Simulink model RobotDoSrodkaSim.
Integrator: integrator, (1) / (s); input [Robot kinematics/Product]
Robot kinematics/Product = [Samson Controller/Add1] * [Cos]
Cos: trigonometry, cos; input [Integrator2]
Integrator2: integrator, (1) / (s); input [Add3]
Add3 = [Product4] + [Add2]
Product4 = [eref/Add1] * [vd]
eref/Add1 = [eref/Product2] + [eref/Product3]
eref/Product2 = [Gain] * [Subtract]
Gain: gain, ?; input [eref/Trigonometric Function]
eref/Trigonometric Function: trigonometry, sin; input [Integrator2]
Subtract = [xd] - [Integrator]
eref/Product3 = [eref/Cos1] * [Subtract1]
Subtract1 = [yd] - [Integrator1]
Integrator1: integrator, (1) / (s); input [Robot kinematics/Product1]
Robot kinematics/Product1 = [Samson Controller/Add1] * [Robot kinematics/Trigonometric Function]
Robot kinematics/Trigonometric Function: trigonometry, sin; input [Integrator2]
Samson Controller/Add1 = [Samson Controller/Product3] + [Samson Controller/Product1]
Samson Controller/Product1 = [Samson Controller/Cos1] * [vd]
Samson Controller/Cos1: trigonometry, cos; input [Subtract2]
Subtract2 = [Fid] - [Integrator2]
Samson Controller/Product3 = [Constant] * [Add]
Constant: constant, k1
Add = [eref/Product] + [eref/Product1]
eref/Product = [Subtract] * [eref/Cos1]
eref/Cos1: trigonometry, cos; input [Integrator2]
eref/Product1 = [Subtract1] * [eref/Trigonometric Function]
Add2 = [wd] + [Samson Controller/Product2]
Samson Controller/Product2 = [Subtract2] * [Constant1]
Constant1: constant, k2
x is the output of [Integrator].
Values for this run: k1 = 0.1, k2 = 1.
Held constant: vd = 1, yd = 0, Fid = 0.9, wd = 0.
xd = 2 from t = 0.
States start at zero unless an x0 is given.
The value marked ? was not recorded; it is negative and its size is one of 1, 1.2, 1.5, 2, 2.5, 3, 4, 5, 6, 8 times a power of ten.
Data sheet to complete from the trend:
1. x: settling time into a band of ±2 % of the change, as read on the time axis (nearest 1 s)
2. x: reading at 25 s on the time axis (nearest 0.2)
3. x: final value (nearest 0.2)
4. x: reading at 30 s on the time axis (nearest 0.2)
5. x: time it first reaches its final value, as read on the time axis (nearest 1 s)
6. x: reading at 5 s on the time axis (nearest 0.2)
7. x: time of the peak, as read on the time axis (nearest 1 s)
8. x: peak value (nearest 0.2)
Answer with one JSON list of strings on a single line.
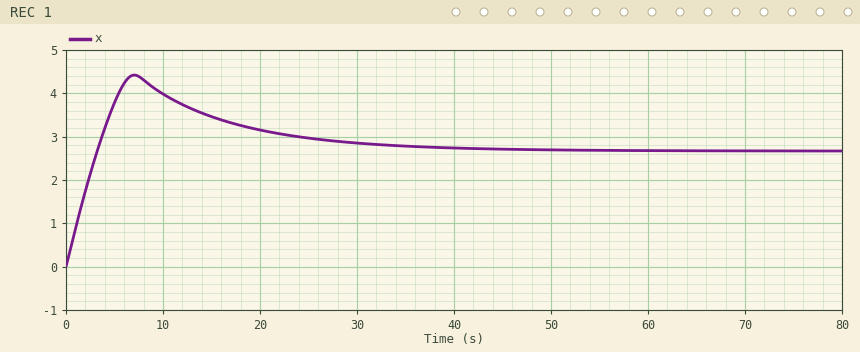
["43 s", "3.0", "2.6", "2.8", "3 s", "3.8", "7 s", "4.4"]
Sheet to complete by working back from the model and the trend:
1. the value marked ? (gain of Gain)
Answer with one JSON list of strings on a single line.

["-0.8"]
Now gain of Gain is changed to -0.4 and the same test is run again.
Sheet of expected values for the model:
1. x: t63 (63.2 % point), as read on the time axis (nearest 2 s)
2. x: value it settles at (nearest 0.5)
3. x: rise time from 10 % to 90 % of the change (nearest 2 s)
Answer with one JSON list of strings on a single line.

["8 s", "7.5", "14 s"]
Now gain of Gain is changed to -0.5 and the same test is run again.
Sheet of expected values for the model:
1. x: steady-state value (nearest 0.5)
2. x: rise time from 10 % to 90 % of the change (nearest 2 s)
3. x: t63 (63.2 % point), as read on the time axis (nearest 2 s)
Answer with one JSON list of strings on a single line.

["6.5", "18 s", "6 s"]
